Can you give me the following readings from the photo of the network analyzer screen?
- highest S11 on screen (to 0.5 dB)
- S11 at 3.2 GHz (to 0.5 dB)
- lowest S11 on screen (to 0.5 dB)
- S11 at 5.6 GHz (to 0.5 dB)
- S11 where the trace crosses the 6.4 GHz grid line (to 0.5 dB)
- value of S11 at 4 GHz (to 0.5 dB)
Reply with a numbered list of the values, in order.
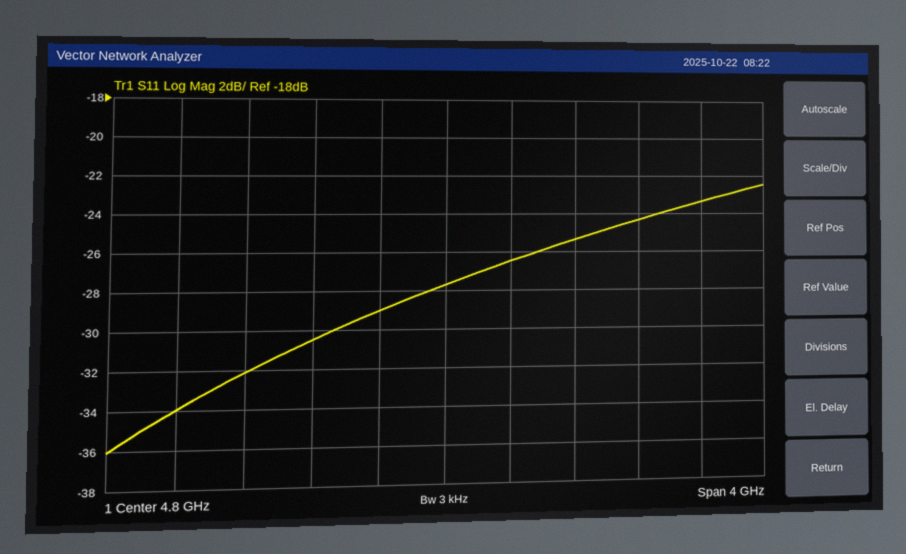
1. -22.5 dB
2. -34.0 dB
3. -36.0 dB
4. -25.5 dB
5. -23.5 dB
6. -30.5 dB
